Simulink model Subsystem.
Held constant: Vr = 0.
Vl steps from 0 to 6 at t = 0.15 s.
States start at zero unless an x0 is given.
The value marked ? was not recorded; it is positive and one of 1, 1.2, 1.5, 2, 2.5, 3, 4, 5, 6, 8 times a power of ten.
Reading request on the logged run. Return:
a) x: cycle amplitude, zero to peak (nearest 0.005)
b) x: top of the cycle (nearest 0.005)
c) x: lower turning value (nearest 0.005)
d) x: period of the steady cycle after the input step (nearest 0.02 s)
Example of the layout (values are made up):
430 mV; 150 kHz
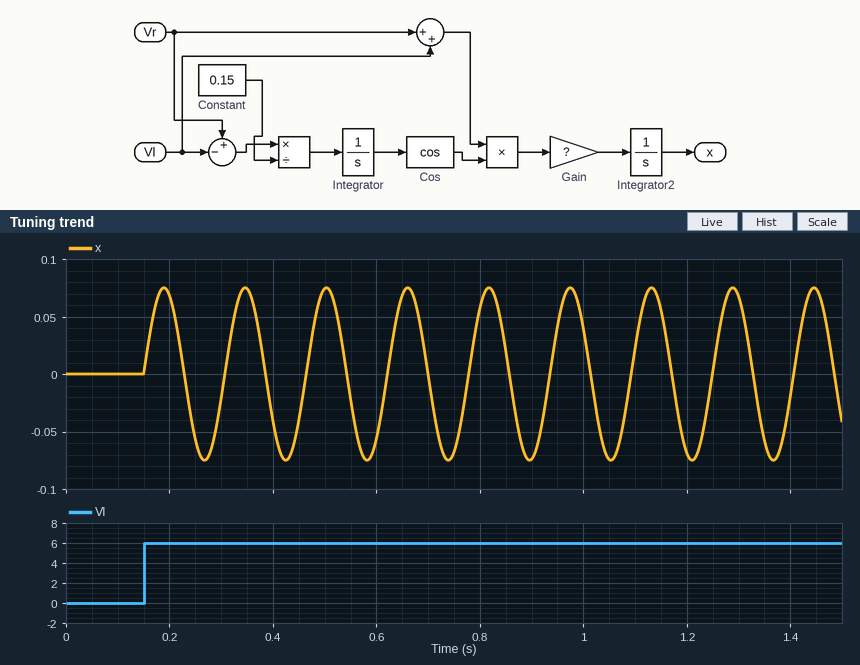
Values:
0.075; 0.075; -0.075; 0.16 s
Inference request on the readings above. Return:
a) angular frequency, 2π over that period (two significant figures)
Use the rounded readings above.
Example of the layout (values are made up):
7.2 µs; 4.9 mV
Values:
39 rad/s
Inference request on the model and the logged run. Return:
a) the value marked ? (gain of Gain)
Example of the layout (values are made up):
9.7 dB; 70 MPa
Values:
0.5
